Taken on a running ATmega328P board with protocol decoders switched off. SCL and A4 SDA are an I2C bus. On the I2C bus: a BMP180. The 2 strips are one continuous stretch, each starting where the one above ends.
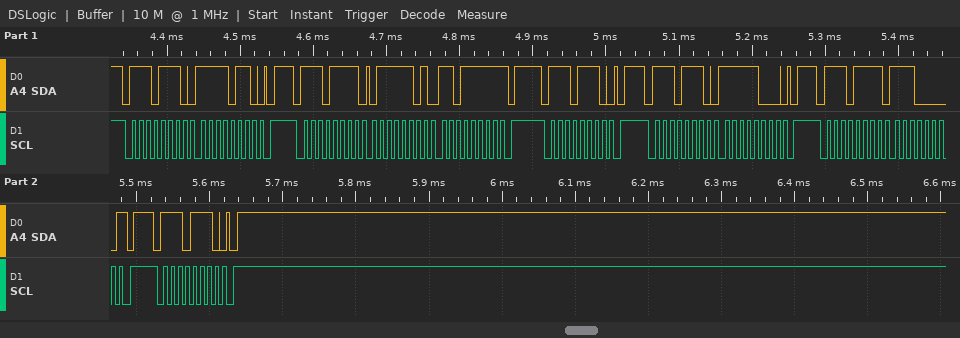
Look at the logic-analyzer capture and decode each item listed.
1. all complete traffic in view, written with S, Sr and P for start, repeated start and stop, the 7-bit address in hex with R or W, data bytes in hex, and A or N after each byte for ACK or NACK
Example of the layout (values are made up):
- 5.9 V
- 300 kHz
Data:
- S 77W A F6 A P S 77R A 7D A DF N P S 77W A P S 77W A F8 A P S 77R A E0 N P S 77W A P
